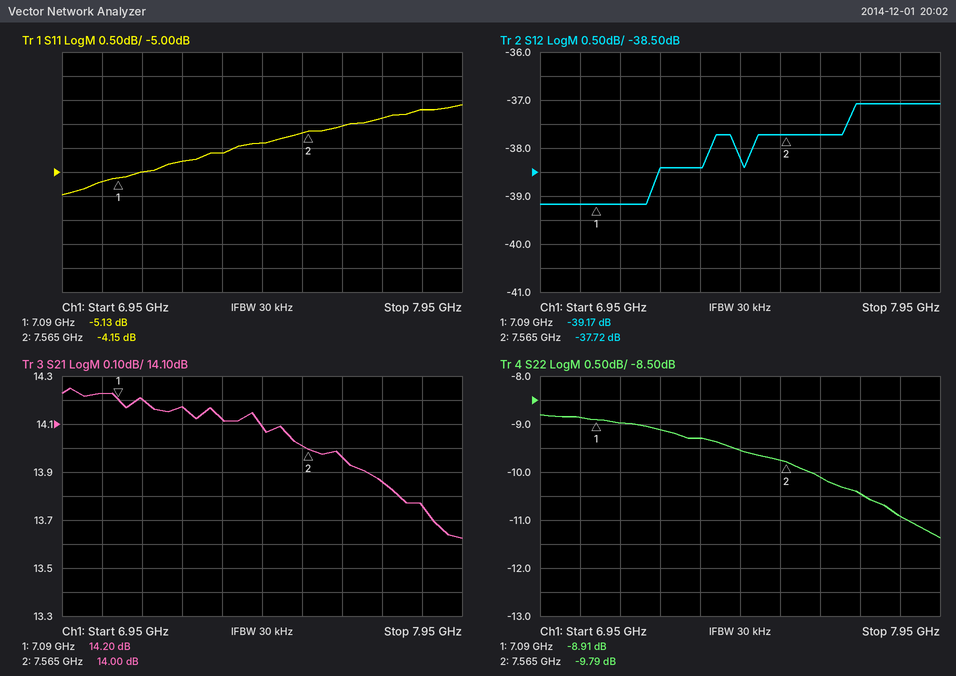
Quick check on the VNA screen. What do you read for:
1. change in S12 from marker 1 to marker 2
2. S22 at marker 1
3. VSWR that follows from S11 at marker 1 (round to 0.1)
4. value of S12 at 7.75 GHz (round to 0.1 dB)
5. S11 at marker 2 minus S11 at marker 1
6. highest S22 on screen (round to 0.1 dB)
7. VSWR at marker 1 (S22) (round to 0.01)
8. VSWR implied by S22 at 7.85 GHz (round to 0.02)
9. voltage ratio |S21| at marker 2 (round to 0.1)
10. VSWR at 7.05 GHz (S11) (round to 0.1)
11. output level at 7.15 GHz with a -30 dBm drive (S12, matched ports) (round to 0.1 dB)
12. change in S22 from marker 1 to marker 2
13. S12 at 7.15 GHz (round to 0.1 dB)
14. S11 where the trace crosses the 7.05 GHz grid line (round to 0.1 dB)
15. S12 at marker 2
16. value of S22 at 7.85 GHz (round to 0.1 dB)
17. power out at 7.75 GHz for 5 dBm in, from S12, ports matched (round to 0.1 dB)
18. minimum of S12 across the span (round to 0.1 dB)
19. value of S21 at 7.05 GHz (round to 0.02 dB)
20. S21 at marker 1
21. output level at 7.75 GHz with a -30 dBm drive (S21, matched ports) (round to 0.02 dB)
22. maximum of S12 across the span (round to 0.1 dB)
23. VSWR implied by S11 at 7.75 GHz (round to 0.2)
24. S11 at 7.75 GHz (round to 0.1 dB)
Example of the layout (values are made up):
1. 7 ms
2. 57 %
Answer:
1. 1.45 dB
2. -8.91 dB
3. 3.5
4. -37.1 dB
5. 0.98 dB
6. -8.8 dB
7. 2.12
8. 1.80
9. 5.0
10. 3.4
11. -69.2 dBm
12. -0.88 dB
13. -39.2 dB
14. -5.2 dB
15. -37.72 dB
16. -10.9 dB
17. -32.1 dBm
18. -39.2 dB
19. 14.22 dB
20. 14.20 dB
21. -16.14 dBm
22. -37.1 dB
23. 4.6
24. -3.9 dB
